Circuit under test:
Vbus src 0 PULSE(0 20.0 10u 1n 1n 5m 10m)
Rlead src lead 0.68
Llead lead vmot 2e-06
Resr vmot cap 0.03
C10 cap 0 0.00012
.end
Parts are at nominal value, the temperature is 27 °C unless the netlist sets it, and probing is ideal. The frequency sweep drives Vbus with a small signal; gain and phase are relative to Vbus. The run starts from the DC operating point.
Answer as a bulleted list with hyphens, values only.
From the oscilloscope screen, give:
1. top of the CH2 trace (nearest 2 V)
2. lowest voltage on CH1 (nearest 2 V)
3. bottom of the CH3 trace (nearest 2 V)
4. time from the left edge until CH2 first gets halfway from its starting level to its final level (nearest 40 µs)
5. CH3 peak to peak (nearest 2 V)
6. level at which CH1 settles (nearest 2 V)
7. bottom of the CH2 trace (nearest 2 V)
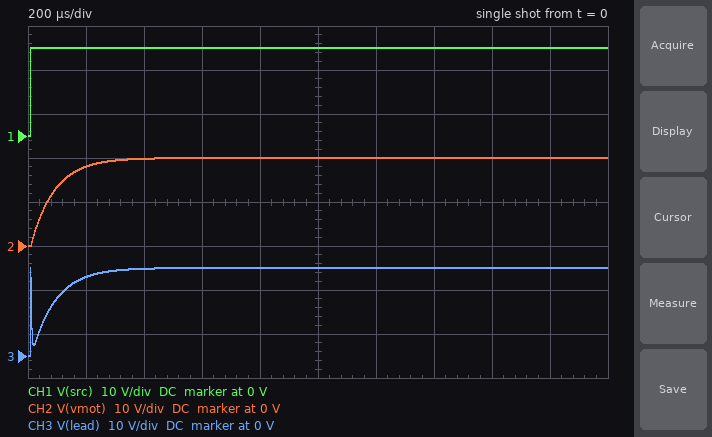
- 20 V
- 0 V
- 0 V
- 80 µs
- 20 V
- 20 V
- 0 V
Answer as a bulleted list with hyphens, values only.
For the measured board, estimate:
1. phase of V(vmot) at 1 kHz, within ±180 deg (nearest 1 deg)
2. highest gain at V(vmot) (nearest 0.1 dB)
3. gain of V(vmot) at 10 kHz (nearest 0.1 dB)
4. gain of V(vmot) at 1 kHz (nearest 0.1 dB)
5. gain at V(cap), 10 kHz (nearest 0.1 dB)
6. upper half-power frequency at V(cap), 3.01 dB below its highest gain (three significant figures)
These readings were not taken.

- -27 deg
- 0 dB
- -14.4 dB
- -1.0 dB
- -14.6 dB
- 1.93 kHz
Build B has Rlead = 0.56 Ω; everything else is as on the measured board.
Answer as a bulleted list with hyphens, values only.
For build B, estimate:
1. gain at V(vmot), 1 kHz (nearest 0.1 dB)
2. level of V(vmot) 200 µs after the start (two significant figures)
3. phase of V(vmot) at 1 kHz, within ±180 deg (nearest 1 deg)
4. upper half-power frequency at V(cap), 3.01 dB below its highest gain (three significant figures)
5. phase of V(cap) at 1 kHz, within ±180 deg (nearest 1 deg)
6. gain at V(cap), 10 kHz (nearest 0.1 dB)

- -0.7 dB
- 19 V
- -23 deg
- 2.36 kHz
- -24 deg
- -13.0 dB
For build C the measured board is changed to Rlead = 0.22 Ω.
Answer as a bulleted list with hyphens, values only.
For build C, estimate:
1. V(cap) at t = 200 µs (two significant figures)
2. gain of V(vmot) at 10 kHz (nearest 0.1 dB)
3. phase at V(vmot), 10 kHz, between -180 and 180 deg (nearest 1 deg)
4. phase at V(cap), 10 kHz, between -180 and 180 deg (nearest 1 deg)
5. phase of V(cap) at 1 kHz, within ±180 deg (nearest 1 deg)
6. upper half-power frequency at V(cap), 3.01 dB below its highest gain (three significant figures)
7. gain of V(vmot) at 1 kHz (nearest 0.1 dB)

- 20 V
- -5.3 dB
- -76 deg
- -88 deg
- -11 deg
- 6.92 kHz
- -0.1 dB
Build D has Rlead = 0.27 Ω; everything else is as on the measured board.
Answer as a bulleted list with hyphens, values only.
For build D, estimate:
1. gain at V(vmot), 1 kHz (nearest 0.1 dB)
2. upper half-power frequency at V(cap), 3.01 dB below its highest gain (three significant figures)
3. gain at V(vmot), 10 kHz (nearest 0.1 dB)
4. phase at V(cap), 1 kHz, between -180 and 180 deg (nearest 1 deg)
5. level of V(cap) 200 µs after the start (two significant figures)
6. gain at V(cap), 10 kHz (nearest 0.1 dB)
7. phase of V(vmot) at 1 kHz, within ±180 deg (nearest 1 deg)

- -0.1 dB
- 5.36 kHz
- -6.9 dB
- -13 deg
- 20 V
- -7.1 dB
- -12 deg
